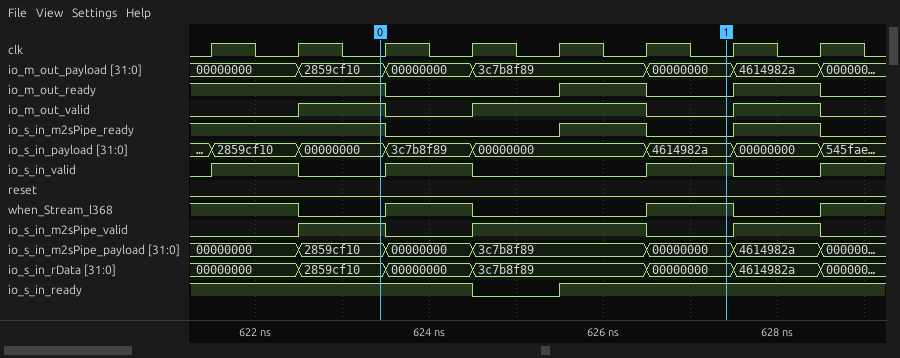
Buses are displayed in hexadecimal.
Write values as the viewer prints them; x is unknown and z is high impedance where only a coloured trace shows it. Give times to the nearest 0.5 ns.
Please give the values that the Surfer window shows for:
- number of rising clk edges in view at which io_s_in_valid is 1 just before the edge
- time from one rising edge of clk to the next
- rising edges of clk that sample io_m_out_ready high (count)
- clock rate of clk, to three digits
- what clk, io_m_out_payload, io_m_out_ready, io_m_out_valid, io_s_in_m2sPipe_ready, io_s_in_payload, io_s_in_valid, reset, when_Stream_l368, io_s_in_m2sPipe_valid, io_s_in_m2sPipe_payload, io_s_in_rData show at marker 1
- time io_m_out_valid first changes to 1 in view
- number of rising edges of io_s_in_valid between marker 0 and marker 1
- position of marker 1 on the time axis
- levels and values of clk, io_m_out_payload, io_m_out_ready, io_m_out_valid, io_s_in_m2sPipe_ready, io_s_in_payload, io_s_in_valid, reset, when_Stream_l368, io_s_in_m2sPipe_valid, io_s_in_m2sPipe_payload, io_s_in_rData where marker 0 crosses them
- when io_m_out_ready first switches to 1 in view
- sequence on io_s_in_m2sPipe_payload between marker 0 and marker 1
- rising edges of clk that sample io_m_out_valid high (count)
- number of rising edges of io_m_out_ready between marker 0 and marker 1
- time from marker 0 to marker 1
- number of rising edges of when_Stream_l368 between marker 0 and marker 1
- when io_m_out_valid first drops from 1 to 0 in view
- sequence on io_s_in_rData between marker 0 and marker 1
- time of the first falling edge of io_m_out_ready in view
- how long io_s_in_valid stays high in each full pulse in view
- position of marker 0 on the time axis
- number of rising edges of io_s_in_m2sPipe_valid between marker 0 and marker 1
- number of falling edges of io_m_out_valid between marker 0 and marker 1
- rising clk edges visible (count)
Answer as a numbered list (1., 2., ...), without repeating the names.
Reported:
1. 3
2. 1 ns
3. 5
4. 1.00 GHz
5. clk=0, io_m_out_payload=00000000, io_m_out_ready=0, io_m_out_valid=0, io_s_in_m2sPipe_ready=0, io_s_in_payload=4614982a, io_s_in_valid=1, reset=0, when_Stream_l368=1, io_s_in_m2sPipe_valid=0, io_s_in_m2sPipe_payload=00000000, io_s_in_rData=00000000
6. 622.5 ns
7. 2
8. 627.5 ns
9. clk=0, io_m_out_payload=2859cf10, io_m_out_ready=1, io_m_out_valid=1, io_s_in_m2sPipe_ready=1, io_s_in_payload=00000000, io_s_in_valid=0, reset=0, when_Stream_l368=0, io_s_in_m2sPipe_valid=1, io_s_in_m2sPipe_payload=2859cf10, io_s_in_rData=2859cf10
10. 625.5 ns
11. 2859cf10, 00000000, 3c7b8f89, 00000000
12. 4
13. 1
14. 4 ns
15. 2
16. 623.5 ns
17. 2859cf10, 00000000, 3c7b8f89, 00000000
18. 623.5 ns
19. 1 ns, 1 ns, 1 ns
20. 623.5 ns
21. 1
22. 2
23. 8
